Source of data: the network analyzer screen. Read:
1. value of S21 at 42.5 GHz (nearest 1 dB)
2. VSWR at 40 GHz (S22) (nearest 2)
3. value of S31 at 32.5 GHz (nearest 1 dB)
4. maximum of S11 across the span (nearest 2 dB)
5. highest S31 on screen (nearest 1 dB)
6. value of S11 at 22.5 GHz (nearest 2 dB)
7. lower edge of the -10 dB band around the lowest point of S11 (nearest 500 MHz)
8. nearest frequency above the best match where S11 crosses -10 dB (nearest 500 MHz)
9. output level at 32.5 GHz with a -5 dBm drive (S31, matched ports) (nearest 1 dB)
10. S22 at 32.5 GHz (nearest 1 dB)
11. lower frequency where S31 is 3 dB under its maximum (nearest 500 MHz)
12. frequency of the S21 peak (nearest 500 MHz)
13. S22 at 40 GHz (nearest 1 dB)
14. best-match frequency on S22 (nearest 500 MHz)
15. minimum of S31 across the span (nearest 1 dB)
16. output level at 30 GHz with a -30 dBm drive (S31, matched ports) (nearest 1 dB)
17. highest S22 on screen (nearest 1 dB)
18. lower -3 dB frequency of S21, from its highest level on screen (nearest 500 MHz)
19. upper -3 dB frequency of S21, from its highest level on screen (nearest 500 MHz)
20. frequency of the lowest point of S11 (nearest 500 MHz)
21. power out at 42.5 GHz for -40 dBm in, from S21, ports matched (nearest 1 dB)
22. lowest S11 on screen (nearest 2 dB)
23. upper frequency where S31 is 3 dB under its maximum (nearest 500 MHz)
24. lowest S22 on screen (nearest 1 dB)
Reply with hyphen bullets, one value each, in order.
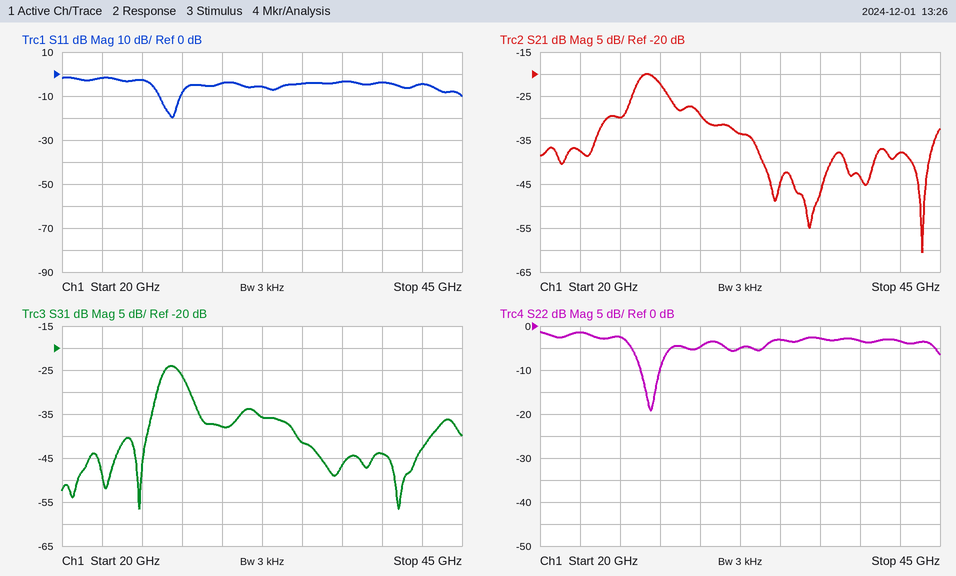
- -38 dB
- 6
- -36 dB
- -2 dB
- -24 dB
- -2 dB
- 26.0 GHz
- 27.5 GHz
- -41 dBm
- -5 dB
- 26.0 GHz
- 26.5 GHz
- -3 dB
- 27.0 GHz
- -57 dB
- -68 dBm
- -1 dB
- 26.0 GHz
- 27.5 GHz
- 27.0 GHz
- -78 dBm
- -20 dB
- 27.5 GHz
- -19 dB
